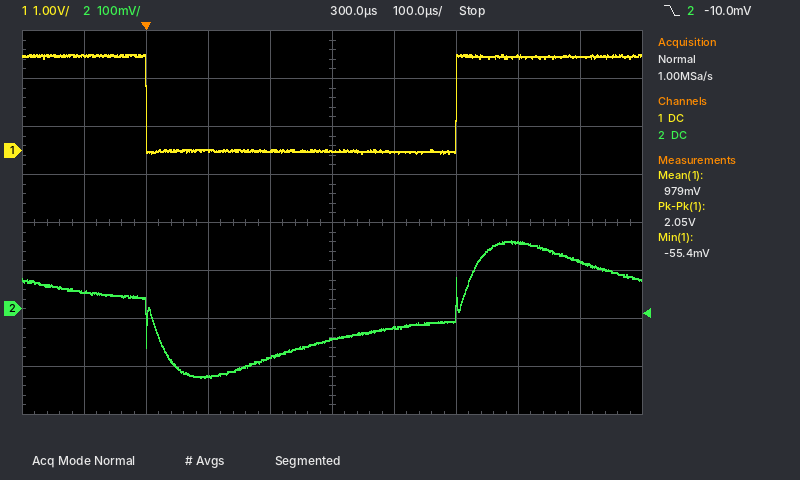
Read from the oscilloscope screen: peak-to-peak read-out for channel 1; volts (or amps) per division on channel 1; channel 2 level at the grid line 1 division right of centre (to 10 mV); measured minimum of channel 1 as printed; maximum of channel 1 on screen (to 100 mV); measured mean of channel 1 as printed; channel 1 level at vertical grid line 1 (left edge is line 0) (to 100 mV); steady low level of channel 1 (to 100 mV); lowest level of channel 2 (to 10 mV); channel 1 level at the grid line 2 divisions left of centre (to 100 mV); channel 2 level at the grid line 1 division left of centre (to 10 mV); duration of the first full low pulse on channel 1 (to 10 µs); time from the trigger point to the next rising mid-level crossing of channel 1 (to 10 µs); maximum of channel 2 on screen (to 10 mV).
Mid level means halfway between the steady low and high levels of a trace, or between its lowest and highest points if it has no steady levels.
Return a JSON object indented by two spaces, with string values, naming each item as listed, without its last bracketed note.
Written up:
{
  "peak-to-peak read-out for channel 1": "2.05 V",
  "volts (or amps) per division on channel 1": "1 V",
  "channel 2 level at the grid line 1 division right of centre": "-40 mV",
  "measured minimum of channel 1 as printed": "-55.4 mV",
  "maximum of channel 1 on screen": "2.0 V",
  "measured mean of channel 1 as printed": "979 mV",
  "channel 1 level at vertical grid line 1 (left edge is line 0)": "2.0 V",
  "steady low level of channel 1": "0.0 V",
  "lowest level of channel 2": "-140 mV",
  "channel 1 level at the grid line 2 divisions left of centre": "0.0 V",
  "channel 2 level at the grid line 1 division left of centre": "-100 mV",
  "duration of the first full low pulse on channel 1": "500 µs",
  "time from the trigger point to the next rising mid-level crossing of channel 1": "500 µs",
  "maximum of channel 2 on screen": "140 mV"
}
